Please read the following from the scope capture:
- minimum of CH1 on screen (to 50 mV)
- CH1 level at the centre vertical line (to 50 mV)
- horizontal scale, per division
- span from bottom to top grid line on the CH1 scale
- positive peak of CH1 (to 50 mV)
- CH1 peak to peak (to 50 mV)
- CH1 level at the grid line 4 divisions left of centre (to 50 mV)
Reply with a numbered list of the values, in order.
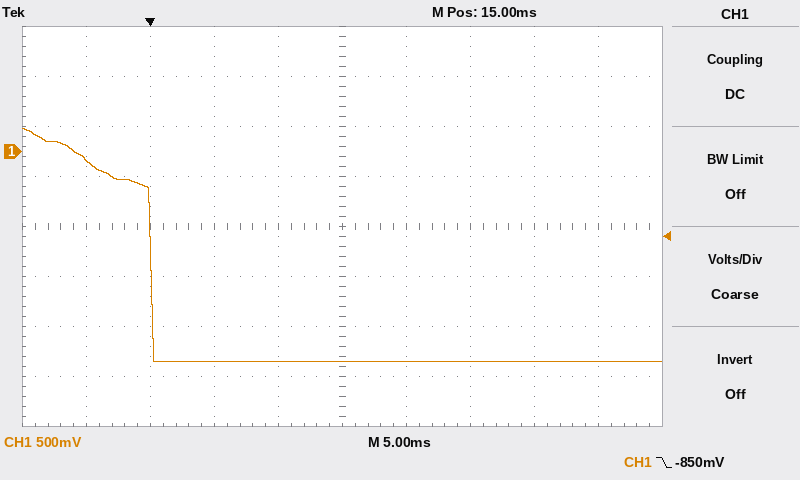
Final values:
1. -2.10 V
2. -2.10 V
3. 5 ms
4. 4 V
5. 250 mV
6. 2.35 V
7. -100 mV
